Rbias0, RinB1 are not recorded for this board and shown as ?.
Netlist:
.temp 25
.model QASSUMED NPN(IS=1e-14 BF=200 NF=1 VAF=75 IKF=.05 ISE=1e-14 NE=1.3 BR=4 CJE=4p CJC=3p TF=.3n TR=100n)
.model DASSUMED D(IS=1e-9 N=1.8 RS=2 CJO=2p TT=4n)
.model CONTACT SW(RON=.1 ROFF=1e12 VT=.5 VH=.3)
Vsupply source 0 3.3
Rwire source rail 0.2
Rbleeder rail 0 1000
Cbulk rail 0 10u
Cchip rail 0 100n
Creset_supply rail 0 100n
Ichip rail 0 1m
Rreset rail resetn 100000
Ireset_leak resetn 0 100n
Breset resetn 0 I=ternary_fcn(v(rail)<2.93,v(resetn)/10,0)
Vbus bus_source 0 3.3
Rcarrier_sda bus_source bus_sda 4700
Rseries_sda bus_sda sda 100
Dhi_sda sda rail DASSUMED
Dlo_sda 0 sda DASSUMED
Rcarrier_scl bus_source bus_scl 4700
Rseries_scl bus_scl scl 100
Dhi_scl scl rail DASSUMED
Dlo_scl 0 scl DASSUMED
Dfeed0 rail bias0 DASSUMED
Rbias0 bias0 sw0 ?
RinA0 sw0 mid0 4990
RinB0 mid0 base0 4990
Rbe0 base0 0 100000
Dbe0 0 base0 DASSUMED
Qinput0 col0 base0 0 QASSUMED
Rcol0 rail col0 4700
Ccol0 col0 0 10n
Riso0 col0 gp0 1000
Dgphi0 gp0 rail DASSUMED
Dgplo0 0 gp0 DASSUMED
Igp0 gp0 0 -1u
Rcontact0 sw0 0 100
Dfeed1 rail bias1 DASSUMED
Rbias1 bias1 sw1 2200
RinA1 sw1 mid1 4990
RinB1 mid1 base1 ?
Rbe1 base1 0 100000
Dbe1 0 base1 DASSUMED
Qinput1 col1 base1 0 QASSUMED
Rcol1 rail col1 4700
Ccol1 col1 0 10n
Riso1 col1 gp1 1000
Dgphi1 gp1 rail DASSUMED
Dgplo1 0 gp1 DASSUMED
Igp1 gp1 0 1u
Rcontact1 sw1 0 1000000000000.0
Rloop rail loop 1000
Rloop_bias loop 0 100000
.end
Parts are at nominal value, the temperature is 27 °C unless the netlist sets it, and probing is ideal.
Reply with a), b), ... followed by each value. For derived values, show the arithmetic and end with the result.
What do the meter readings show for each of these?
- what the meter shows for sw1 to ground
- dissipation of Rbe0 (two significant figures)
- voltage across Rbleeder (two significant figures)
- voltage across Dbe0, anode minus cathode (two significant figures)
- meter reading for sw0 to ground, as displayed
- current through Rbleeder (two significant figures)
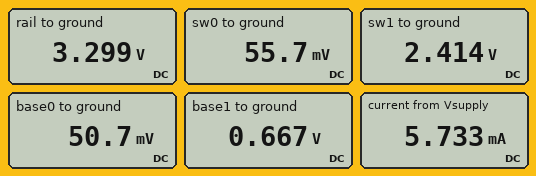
a) 2.414 V
b) (50.7 mV)^2 / 100 kΩ = 26 nW
c) 3.299 V = 3.3 V
d) 0 V - 50.7 mV = -51 mV
e) 55.7 mV
f) (3.299 V) / 1 kΩ = 3.3 mA
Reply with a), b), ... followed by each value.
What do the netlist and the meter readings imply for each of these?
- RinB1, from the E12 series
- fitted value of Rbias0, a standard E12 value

a) 6.8 kΩ
b) 4.7 kΩ
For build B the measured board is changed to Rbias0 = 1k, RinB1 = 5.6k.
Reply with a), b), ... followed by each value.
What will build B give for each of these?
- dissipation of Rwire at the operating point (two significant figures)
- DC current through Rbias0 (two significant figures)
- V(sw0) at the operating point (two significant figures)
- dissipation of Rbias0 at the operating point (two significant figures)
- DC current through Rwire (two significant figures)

a) 11 µW
b) 2.4 mA
c) 240 mV
d) 5.6 mW
e) 7.6 mA
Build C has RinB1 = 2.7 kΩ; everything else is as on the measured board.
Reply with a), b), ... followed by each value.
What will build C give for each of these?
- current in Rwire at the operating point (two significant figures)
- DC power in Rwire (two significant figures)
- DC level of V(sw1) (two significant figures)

a) 5.8 mA
b) 6.7 µW
c) 2.3 V
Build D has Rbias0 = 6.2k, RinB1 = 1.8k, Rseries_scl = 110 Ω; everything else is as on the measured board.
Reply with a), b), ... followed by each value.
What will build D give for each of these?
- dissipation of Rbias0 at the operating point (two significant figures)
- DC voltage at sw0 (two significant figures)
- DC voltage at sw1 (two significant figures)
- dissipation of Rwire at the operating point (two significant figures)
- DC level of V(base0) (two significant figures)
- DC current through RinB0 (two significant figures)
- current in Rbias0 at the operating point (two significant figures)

a) 1.1 mW
b) 43 mV
c) 2.2 V
d) 6.5 µW
e) 39 mV
f) 390 nA
g) 430 µA
